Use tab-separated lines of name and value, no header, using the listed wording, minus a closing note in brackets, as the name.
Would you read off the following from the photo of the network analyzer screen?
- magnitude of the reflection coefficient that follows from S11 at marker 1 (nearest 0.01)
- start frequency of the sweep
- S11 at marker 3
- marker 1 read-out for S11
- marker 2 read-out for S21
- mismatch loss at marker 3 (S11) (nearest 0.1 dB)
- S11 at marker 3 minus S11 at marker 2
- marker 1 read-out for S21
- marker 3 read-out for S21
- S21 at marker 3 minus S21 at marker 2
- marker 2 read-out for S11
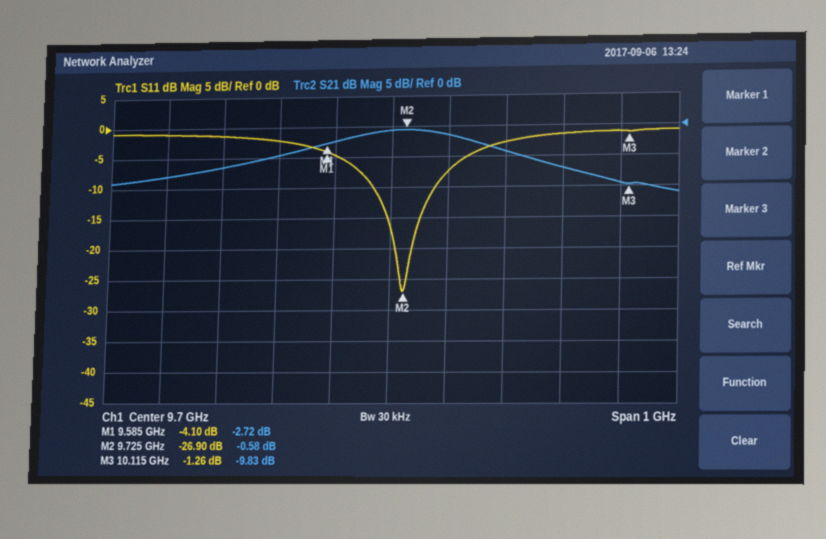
magnitude of the reflection coefficient that follows from S11 at marker 1	0.62
start frequency of the sweep	9.2 GHz
S11 at marker 3	-1.26 dB
marker 1 read-out for S11	-4.10 dB
marker 2 read-out for S21	-0.58 dB
mismatch loss at marker 3 (S11)	6.0 dB
S11 at marker 3 minus S11 at marker 2	25.64 dB
marker 1 read-out for S21	-2.72 dB
marker 3 read-out for S21	-9.83 dB
S21 at marker 3 minus S21 at marker 2	-9.25 dB
marker 2 read-out for S11	-26.90 dB
